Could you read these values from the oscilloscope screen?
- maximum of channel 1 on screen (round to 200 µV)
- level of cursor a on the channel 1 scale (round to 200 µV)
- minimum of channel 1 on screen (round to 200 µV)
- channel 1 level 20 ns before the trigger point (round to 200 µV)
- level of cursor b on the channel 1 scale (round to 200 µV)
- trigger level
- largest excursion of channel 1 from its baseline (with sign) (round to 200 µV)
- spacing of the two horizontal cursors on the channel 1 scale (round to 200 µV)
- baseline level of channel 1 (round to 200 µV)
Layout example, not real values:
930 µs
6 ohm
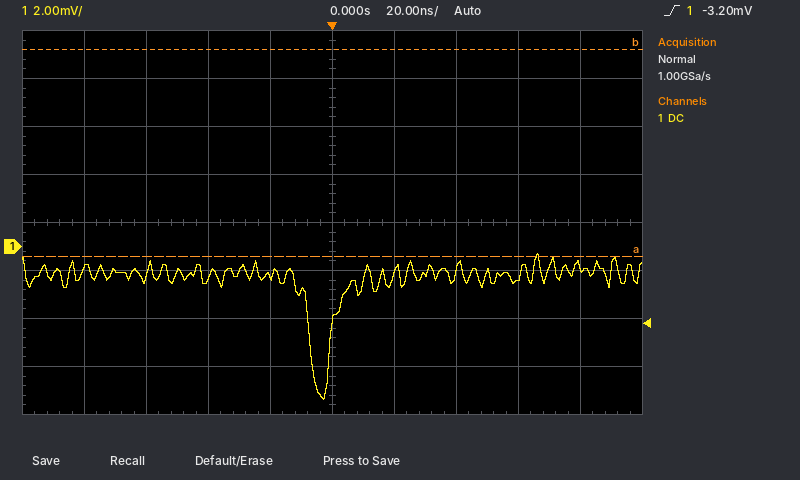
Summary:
-200 µV
-400 µV
-6.4 mV
-1.2 mV
8.2 mV
-3.20 mV
-5.2 mV
8.6 mV
-1.2 mV
